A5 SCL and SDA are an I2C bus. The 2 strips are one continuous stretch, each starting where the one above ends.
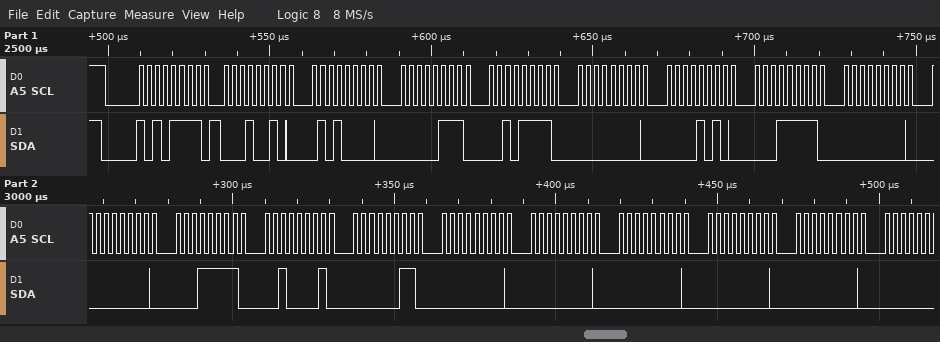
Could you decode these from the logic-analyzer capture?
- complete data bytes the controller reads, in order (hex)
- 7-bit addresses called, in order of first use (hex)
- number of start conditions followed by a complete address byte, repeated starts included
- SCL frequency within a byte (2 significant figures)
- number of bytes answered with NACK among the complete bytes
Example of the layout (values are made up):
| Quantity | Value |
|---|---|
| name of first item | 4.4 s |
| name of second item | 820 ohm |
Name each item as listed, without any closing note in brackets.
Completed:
| Quantity | Value |
|---|---|
| complete data bytes the controller reads, in order | 12 50 07 2F 00 0A 1F 00 00 1F 21 03 00 00 00 00 00 |
| 7-bit addresses called, in order of first use | 0x57 |
| number of start conditions followed by a complete address byte, repeated starts included | 1 |
| SCL frequency within a byte | 400 kHz |
| number of bytes answered with NACK among the complete bytes | 0 |
